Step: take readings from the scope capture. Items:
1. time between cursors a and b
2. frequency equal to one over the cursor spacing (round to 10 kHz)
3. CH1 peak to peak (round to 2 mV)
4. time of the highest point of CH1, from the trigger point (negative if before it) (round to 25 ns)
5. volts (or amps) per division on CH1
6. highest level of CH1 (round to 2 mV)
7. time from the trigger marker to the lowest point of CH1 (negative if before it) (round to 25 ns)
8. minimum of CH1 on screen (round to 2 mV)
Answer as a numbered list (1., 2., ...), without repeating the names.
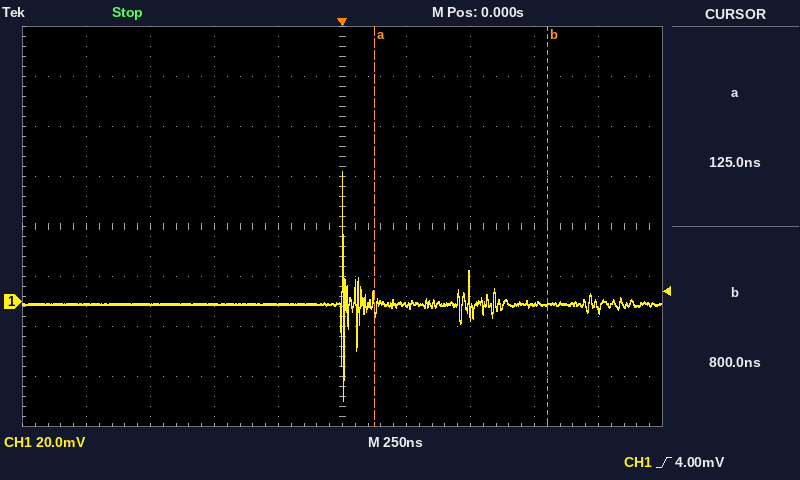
1. 675 ns
2. 1.48 MHz
3. 92 mV
4. 0 ns
5. 20 mV
6. 52 mV
7. 0 ns
8. -40 mV
